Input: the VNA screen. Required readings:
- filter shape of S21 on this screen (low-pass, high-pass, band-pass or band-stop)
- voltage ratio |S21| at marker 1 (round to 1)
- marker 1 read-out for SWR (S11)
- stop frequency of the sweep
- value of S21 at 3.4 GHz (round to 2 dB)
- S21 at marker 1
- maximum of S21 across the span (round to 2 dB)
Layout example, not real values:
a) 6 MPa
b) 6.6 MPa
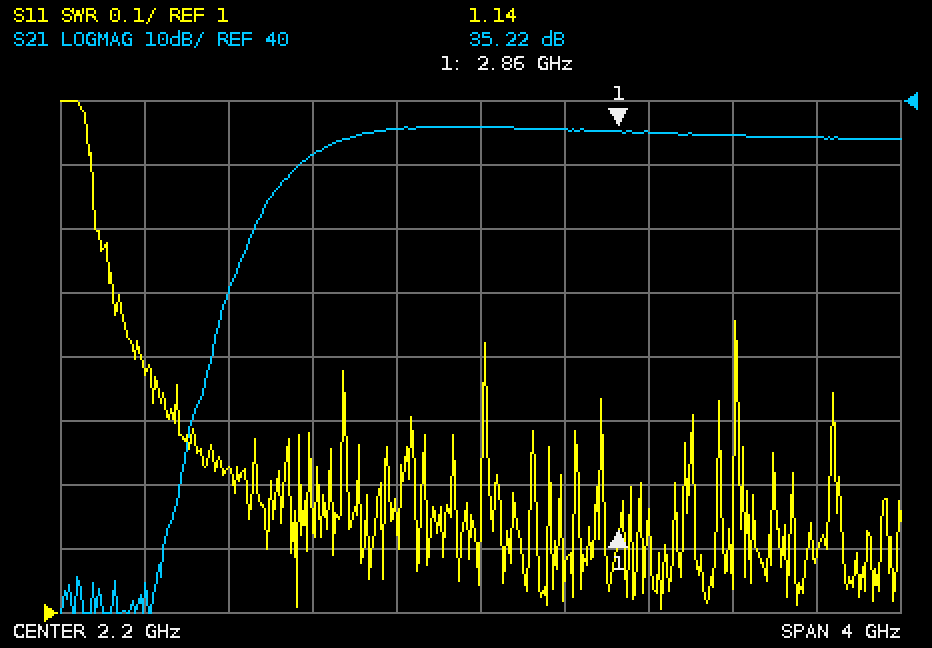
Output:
a) high-pass
b) 58
c) 1.14
d) 4.2 GHz
e) 34 dB
f) 35.22 dB
g) 36 dB
